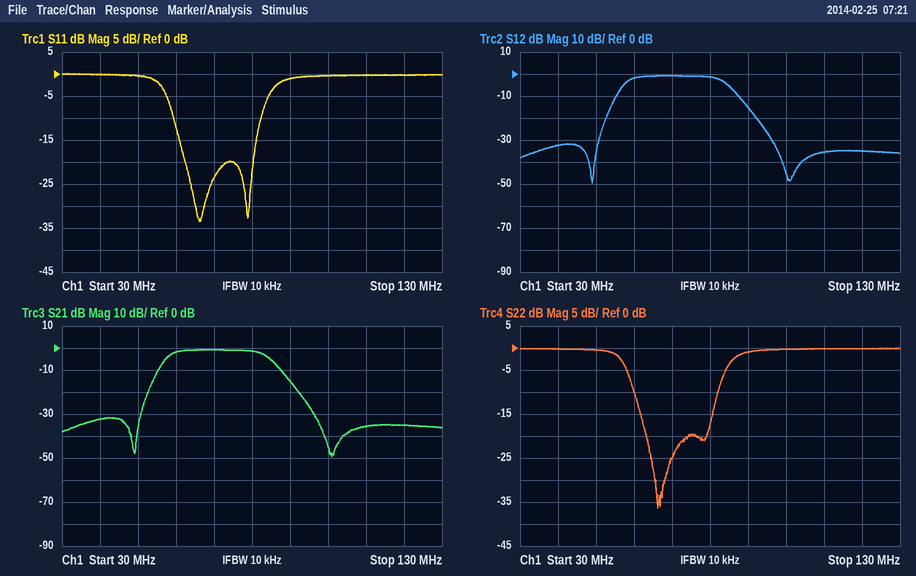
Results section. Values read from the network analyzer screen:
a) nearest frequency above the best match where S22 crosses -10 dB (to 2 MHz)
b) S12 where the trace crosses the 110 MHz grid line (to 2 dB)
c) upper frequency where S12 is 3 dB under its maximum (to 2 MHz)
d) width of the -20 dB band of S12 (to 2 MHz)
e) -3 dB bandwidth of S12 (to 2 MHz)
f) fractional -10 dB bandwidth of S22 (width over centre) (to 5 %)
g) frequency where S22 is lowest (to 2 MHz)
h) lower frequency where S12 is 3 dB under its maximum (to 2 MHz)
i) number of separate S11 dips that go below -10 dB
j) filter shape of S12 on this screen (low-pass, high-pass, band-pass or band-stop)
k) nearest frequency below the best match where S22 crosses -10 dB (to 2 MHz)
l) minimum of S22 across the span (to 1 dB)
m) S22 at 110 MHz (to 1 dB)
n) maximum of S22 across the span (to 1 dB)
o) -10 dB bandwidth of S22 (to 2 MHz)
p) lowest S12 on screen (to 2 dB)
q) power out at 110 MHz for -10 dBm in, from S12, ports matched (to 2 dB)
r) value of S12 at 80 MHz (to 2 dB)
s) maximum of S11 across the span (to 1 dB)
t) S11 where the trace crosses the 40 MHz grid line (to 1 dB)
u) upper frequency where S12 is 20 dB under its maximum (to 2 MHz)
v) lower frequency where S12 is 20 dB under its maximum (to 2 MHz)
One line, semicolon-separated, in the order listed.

82 MHz; -36 dB; 84 MHz; 40 MHz; 26 MHz; 30 %; 66 MHz; 58 MHz; 2; band-pass; 60 MHz; -36 dB; 0 dB; 0 dB; 22 MHz; -50 dB; -46 dBm; -2 dB; 0 dB; 0 dB; 92 MHz; 52 MHz
